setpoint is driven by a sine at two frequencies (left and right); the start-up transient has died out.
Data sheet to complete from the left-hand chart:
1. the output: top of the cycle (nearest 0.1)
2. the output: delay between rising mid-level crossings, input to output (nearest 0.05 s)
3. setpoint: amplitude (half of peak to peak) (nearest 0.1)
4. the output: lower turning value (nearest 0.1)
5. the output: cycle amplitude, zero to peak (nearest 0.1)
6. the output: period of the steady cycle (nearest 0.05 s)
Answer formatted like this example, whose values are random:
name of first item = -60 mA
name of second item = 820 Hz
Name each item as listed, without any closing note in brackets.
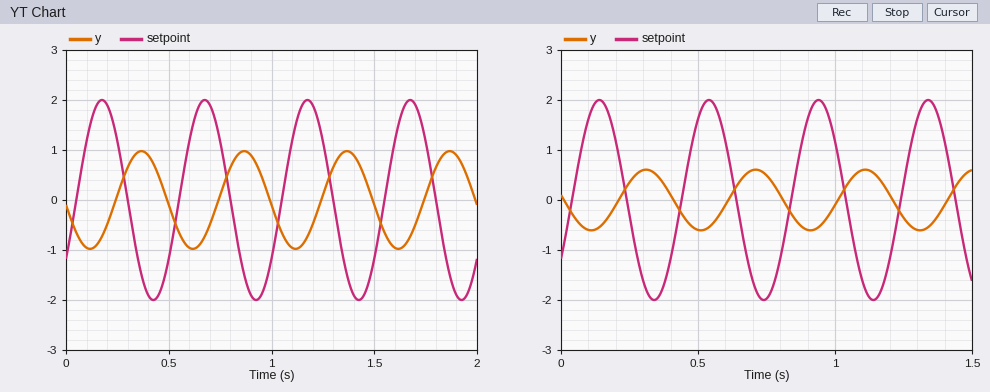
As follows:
the output: top of the cycle = 1.0
the output: delay between rising mid-level crossings, input to output = 0.20 s
setpoint: amplitude (half of peak to peak) = 2.0
the output: lower turning value = -1.0
the output: cycle amplitude, zero to peak = 1.0
the output: period of the steady cycle = 0.50 s
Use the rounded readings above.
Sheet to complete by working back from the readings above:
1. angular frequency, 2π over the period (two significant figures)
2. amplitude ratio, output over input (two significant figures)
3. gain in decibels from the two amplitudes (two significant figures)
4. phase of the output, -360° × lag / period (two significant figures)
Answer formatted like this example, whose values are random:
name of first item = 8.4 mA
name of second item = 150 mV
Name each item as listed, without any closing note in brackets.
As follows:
angular frequency, 2π over the period = 13 rad/s
amplitude ratio, output over input = 0.50
gain in decibels from the two amplitudes = -6.0 dB
phase of the output, -360° × lag / period = -140°
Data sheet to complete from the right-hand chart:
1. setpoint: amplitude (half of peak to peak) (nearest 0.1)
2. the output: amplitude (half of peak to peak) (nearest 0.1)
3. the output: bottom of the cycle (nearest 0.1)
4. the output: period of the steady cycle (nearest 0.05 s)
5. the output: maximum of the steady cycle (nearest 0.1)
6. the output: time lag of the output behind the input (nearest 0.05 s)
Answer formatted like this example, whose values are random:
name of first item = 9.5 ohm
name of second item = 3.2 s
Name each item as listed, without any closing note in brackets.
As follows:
setpoint: amplitude (half of peak to peak) = 2.0
the output: amplitude (half of peak to peak) = 0.6
the output: bottom of the cycle = -0.6
the output: period of the steady cycle = 0.40 s
the output: maximum of the steady cycle = 0.6
the output: time lag of the output behind the input = 0.15 s
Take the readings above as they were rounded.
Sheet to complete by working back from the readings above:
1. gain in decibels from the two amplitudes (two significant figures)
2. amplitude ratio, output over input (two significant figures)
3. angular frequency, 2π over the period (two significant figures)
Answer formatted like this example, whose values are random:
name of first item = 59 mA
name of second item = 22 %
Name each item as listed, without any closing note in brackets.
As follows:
gain in decibels from the two amplitudes = -10 dB
amplitude ratio, output over input = 0.30
angular frequency, 2π over the period = 16 rad/s
